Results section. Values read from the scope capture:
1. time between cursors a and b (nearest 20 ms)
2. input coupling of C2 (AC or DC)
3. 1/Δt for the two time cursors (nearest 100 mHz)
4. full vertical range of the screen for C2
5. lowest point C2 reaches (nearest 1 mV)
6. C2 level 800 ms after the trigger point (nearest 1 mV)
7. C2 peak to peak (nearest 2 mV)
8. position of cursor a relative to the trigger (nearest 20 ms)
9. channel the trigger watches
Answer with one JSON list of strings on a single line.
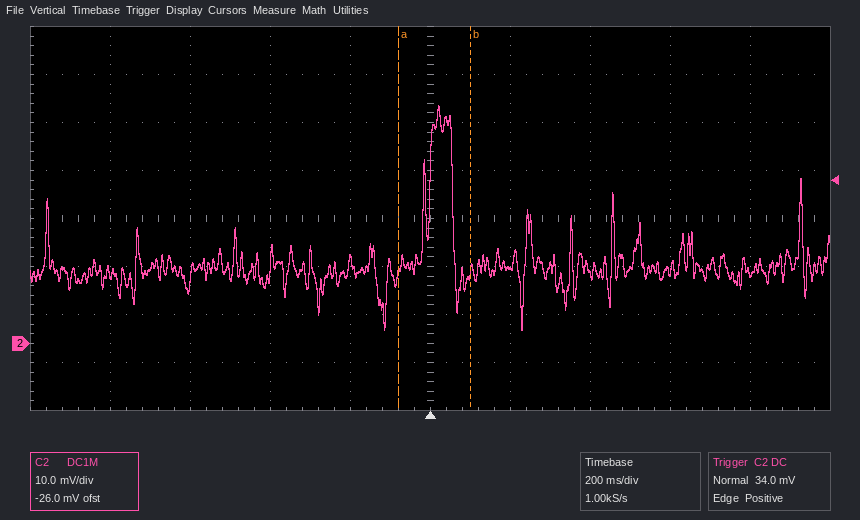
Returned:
["180 ms", "DC", "5.6 Hz", "80 mV", "3 mV", "15 mV", "46 mV", "-80 ms", "C2"]
